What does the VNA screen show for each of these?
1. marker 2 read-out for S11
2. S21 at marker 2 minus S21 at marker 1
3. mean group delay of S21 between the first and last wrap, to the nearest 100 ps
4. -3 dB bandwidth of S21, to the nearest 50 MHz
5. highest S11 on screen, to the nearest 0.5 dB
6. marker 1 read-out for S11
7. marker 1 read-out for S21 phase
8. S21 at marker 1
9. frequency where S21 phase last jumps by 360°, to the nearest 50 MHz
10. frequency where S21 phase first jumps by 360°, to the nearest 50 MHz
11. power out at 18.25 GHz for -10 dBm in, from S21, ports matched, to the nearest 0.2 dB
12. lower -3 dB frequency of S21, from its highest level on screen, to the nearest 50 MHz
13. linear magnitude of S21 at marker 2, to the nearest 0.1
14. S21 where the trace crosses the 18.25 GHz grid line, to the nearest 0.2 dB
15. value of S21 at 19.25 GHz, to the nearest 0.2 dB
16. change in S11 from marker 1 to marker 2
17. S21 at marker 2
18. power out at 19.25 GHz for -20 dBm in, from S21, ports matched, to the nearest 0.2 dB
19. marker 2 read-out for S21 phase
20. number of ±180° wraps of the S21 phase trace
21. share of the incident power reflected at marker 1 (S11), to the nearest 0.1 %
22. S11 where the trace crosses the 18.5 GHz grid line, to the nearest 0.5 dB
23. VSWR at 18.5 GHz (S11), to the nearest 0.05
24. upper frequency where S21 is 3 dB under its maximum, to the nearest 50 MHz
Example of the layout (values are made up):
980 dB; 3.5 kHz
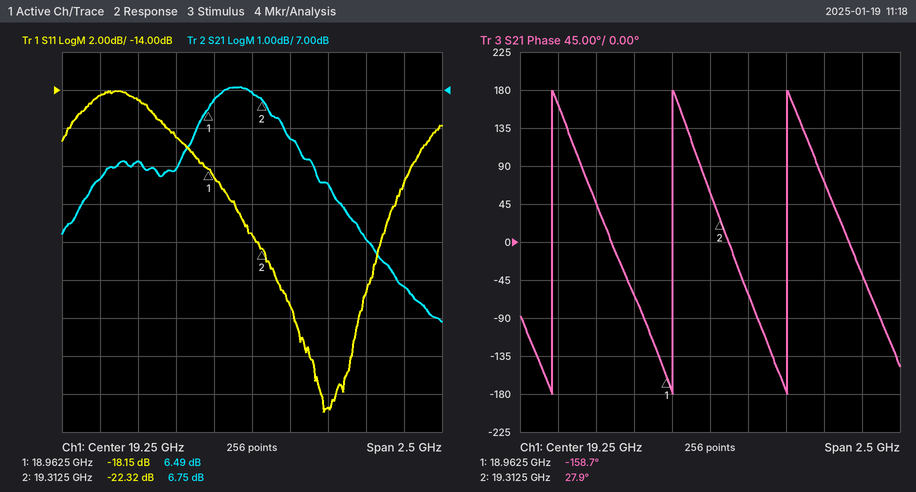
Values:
-22.32 dB; 0.26 dB; 1.3 ns; 1.65 GHz; -14.0 dB; -18.15 dB; -158.7°; 6.49 dB; 19.75 GHz; 18.20 GHz; -5.4 dBm; 18.15 GHz; 2.2; 4.6 dB; 7.0 dB; -4.17 dB; 6.75 dB; -13.0 dBm; 27.9°; 3; 1.5 %; -14.5 dB; 1.45; 19.80 GHz
